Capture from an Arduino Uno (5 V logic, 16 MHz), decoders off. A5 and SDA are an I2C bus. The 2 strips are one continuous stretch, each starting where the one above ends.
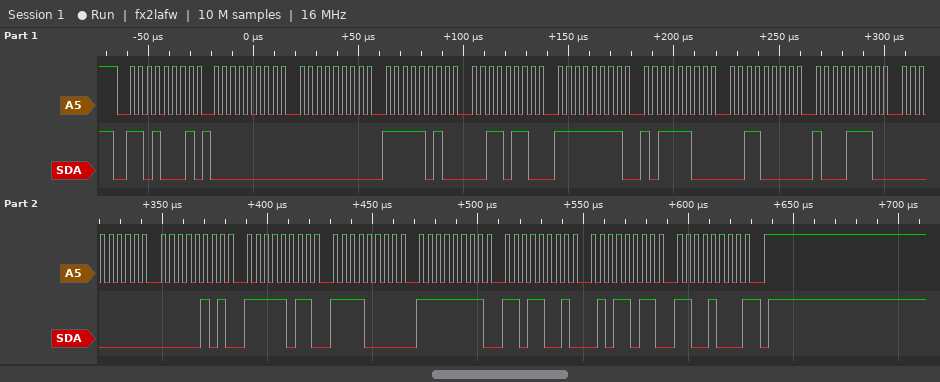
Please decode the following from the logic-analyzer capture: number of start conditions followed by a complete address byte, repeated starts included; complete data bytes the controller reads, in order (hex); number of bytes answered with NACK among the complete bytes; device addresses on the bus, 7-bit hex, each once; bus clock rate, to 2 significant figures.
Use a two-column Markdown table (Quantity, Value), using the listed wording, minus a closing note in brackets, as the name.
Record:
| Quantity | Value |
|---|---|
| number of start conditions followed by a complete address byte, repeated starts included | 1 |
| complete data bytes the controller reads, in order | 00 00 FA 36 FF BC 30 8E 00 05 FB F0 FF D9 5B C8 |
| number of bytes answered with NACK among the complete bytes | 1 |
| device addresses on the bus, 7-bit hex, each once | 0x68 |
| bus clock rate, to 2 significant figures | 250 kHz |
